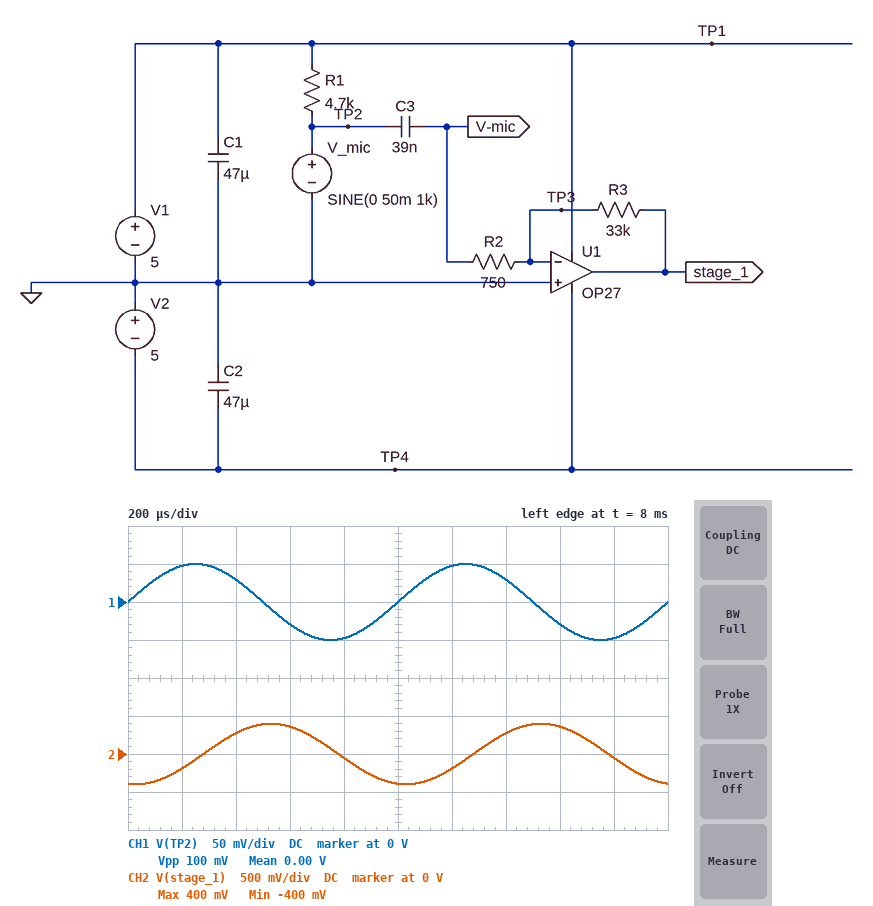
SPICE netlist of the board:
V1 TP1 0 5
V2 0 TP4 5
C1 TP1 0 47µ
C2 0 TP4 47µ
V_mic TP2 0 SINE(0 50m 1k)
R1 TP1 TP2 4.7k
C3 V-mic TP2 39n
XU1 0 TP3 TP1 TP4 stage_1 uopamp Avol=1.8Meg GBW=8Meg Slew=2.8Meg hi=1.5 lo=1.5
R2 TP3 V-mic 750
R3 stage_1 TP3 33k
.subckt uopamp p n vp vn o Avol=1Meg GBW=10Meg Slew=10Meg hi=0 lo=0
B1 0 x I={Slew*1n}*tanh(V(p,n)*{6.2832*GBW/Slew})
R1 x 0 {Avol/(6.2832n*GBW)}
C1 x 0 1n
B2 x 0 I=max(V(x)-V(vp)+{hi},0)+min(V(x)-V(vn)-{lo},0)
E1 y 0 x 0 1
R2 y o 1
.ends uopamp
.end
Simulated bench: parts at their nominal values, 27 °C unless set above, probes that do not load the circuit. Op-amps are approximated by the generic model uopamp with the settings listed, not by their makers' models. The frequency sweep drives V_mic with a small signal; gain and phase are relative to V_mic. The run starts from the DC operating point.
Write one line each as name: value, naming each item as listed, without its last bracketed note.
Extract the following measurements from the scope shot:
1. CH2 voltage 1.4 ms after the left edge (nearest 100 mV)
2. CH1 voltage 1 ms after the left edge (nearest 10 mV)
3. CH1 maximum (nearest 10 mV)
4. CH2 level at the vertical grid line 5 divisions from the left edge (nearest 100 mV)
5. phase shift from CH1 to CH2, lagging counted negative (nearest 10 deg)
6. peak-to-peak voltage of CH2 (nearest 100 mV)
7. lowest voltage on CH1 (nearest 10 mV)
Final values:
CH2 voltage 1.4 ms after the left edge: 300 mV
CH1 voltage 1 ms after the left edge: 0 V
CH1 maximum: 50 mV
CH2 level at the vertical grid line 5 divisions from the left edge: -400 mV
phase shift from CH1 to CH2, lagging counted negative: -100 deg
peak-to-peak voltage of CH2: 800 mV
lowest voltage on CH1: -50 mV
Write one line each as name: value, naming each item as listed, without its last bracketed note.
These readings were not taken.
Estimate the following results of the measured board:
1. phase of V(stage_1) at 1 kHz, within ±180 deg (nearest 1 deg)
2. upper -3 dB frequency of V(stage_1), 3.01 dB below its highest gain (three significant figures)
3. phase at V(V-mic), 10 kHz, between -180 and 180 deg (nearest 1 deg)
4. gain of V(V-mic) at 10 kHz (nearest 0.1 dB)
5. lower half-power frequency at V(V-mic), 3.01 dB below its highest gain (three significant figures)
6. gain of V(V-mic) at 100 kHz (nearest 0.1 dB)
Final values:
phase of V(stage_1) at 1 kHz, within ±180 deg: -100 deg
upper -3 dB frequency of V(stage_1), 3.01 dB below its highest gain: 183 kHz
phase at V(V-mic), 10 kHz, between -180 and 180 deg: 29 deg
gain of V(V-mic) at 10 kHz: -0.9 dB
lower half-power frequency at V(V-mic), 3.01 dB below its highest gain: 5.53 kHz
gain of V(V-mic) at 100 kHz: 0.2 dB
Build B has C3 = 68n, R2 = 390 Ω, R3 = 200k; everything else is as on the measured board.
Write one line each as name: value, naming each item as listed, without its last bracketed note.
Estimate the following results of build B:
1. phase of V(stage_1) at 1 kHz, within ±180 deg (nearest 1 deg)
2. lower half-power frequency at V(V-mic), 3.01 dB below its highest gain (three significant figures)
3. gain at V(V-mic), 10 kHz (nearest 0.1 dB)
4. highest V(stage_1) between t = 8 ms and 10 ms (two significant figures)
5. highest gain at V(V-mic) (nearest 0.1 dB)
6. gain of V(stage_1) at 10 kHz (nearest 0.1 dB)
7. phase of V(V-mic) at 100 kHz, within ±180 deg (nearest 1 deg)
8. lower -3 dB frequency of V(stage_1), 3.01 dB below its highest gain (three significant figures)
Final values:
phase of V(stage_1) at 1 kHz, within ±180 deg: -100 deg
lower half-power frequency at V(V-mic), 3.01 dB below its highest gain: 5.58 kHz
gain at V(V-mic), 10 kHz: 1.5 dB
highest V(stage_1) between t = 8 ms and 10 ms: 3.5 V
highest gain at V(V-mic): 1.7 dB
gain of V(stage_1) at 10 kHz: 54.2 dB
phase of V(V-mic) at 100 kHz, within ±180 deg: 0 deg
lower -3 dB frequency of V(stage_1), 3.01 dB below its highest gain: 4.62 kHz
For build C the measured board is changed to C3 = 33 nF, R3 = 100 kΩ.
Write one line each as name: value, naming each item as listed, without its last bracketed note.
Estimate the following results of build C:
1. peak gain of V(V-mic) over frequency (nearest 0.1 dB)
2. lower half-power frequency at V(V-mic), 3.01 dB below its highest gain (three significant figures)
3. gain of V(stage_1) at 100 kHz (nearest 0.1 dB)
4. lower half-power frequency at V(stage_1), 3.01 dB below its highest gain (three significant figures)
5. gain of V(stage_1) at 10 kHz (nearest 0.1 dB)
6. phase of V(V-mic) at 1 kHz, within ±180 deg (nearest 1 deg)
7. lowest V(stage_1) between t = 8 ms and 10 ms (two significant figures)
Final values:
peak gain of V(V-mic) over frequency: 0.6 dB
lower half-power frequency at V(V-mic), 3.01 dB below its highest gain: 6.59 kHz
gain of V(stage_1) at 100 kHz: 36.9 dB
lower half-power frequency at V(stage_1), 3.01 dB below its highest gain: 5.85 kHz
gain of V(stage_1) at 10 kHz: 41.6 dB
phase of V(V-mic) at 1 kHz, within ±180 deg: 82 deg
lowest V(stage_1) between t = 8 ms and 10 ms: -1.0 V
